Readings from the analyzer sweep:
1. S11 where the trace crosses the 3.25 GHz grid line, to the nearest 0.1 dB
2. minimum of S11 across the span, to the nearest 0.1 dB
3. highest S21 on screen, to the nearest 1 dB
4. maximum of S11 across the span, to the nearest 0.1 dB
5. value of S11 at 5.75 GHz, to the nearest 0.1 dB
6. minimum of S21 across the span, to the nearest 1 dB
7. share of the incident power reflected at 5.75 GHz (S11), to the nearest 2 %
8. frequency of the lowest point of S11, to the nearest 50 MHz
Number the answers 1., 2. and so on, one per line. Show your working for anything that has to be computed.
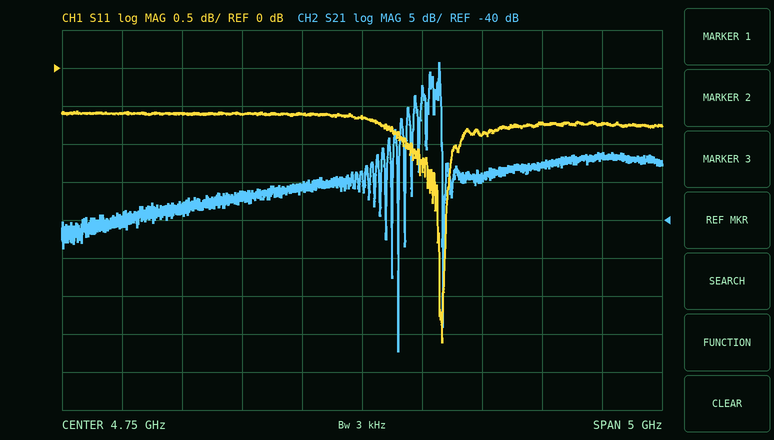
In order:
1. -0.6 dB
2. -3.6 dB
3. -19 dB
4. -0.6 dB
5. -0.9 dB
6. -57 dB
7. 10^(-0.9/10) ≈ 81.3 %, so 82 % to the nearest 2 %
8. 5.40 GHz
